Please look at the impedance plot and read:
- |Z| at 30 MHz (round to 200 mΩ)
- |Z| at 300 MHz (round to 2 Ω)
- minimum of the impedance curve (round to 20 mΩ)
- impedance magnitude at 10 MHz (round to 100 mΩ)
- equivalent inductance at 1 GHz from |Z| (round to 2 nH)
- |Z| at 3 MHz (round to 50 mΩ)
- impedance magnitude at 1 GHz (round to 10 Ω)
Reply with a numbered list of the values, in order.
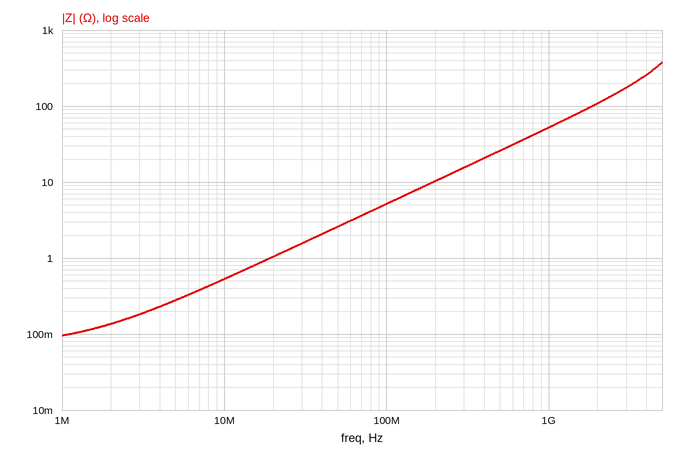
1. 1.6 Ω
2. 16 Ω
3. 100 mΩ
4. 500 mΩ
5. 8 nH
6. 200 mΩ
7. 50 Ω
